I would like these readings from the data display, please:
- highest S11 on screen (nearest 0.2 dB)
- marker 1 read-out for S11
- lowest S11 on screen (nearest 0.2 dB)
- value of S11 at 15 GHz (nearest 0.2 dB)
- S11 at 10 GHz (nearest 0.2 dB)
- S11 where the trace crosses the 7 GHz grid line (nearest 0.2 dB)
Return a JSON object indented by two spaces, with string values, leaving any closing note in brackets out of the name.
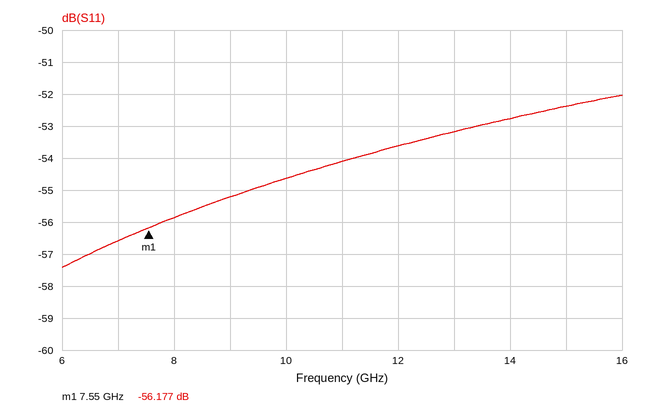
{
  "highest S11 on screen": "-52.0 dB",
  "marker 1 read-out for S11": "-56.177 dB",
  "lowest S11 on screen": "-57.4 dB",
  "value of S11 at 15 GHz": "-52.4 dB",
  "S11 at 10 GHz": "-54.6 dB",
  "S11 where the trace crosses the 7 GHz grid line": "-56.6 dB"
}
